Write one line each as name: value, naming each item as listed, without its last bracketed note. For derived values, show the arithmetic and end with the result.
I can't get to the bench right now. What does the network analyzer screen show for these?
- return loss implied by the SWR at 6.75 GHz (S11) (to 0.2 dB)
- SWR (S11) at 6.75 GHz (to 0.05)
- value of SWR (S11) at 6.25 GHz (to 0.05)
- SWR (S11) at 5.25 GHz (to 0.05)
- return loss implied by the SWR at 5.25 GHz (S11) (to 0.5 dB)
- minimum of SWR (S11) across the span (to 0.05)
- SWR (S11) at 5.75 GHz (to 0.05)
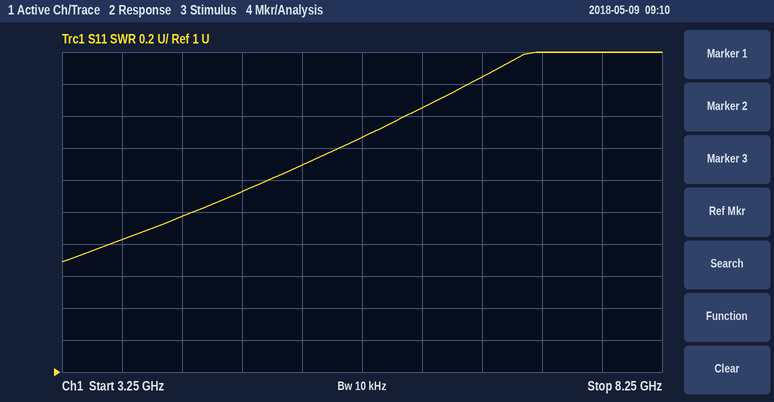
return loss implied by the SWR at 6.75 GHz (S11): −20 log10((2.85 − 1)/(2.85 + 1)) ≈ 6.4 dB
SWR (S11) at 6.75 GHz: 2.85
value of SWR (S11) at 6.25 GHz: 2.65
SWR (S11) at 5.25 GHz: 2.30
return loss implied by the SWR at 5.25 GHz (S11): −20 log10((2.3 − 1)/(2.3 + 1)) ≈ 8.09 dB, so 8.0 dB to the nearest 0.5 dB
minimum of SWR (S11) across the span: 1.70
SWR (S11) at 5.75 GHz: 2.45
